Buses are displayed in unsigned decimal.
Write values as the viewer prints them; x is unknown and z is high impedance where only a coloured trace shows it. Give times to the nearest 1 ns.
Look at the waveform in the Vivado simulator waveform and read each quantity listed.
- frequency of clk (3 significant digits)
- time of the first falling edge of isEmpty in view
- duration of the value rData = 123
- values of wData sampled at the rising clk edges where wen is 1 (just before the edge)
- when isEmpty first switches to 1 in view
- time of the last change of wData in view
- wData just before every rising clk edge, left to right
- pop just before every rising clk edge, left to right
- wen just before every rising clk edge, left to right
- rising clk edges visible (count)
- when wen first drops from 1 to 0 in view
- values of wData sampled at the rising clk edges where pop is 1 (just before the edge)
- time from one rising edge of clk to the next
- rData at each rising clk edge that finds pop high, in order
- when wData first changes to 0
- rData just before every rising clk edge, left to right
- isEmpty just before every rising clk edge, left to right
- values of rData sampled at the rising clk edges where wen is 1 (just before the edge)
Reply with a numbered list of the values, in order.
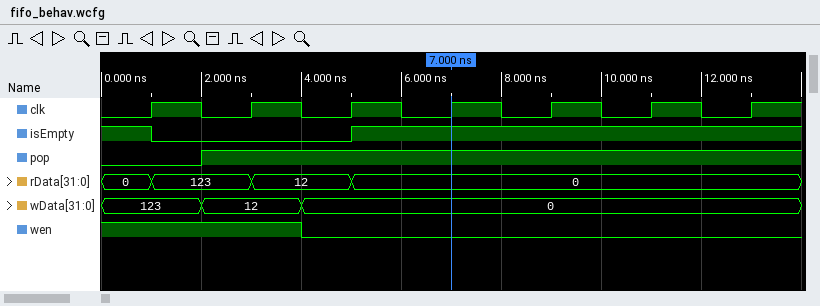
1. 500 MHz
2. 1 ns
3. 2 ns
4. 123, 12
5. 5 ns
6. 4 ns
7. 123, 12, 0, 0, 0, 0, 0
8. 0 1 1 1 1 1 1
9. 1 1 0 0 0 0 0
10. 7
11. 4 ns
12. 12, 0, 0, 0, 0, 0
13. 2 ns
14. 123, 12, 0, 0, 0, 0
15. 4 ns
16. 0, 123, 12, 0, 0, 0, 0
17. 1 0 0 1 1 1 1
18. 0, 123
